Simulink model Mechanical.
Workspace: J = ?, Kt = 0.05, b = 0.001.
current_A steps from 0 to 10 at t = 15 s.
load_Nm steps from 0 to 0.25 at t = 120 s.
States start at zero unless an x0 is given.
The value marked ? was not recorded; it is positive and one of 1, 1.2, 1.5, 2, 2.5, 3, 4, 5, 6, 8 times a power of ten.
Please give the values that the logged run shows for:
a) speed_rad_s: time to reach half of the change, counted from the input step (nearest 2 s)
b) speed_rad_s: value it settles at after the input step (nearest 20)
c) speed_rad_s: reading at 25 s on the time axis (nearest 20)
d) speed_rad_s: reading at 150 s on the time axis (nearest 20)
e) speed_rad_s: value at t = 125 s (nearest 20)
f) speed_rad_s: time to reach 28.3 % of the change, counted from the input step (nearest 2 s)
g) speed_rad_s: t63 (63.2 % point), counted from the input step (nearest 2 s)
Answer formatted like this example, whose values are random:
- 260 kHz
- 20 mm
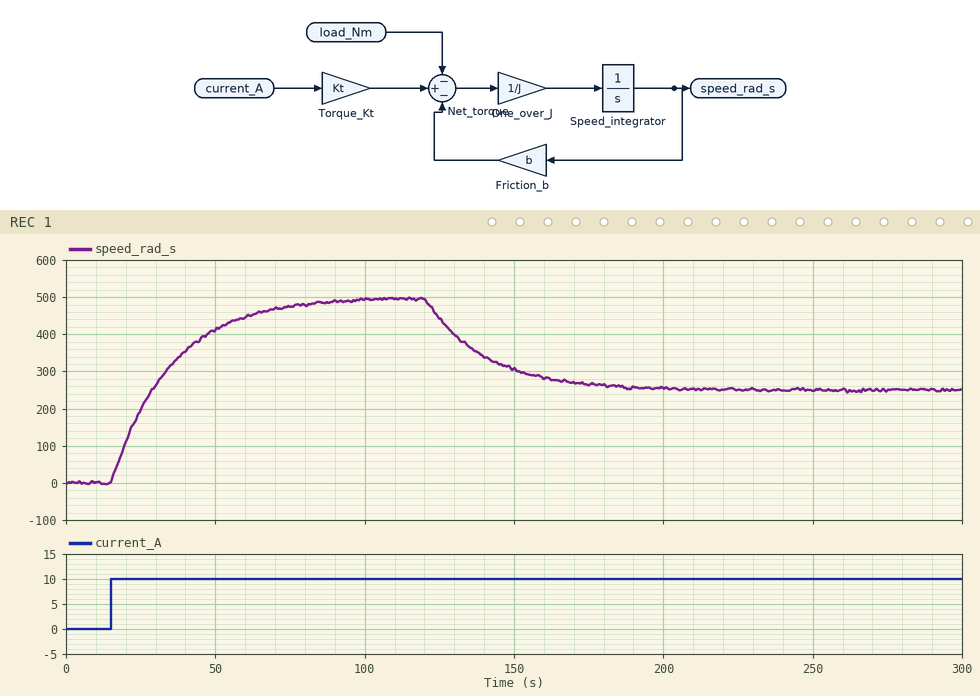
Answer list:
- 14 s
- 500
- 200
- 300
- 440
- 6 s
- 20 s
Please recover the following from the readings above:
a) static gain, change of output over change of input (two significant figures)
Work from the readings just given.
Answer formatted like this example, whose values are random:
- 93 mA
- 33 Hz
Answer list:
- 50
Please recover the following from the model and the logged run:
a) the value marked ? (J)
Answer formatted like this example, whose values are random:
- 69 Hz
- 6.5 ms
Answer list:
- 0.02
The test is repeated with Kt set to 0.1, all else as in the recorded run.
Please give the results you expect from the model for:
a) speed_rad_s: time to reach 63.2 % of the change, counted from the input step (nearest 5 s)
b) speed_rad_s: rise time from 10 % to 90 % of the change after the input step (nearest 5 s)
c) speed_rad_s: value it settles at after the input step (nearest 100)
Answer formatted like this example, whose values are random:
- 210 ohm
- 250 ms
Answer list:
- 20 s
- 45 s
- 1000
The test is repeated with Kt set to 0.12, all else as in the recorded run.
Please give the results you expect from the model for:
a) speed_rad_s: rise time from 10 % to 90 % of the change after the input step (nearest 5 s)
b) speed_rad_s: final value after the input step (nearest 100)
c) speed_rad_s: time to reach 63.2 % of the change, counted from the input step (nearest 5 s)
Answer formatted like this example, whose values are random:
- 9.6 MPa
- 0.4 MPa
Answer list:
- 45 s
- 1200
- 20 s
